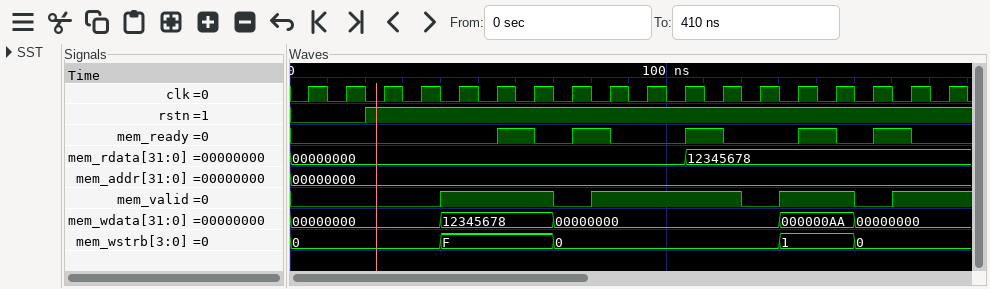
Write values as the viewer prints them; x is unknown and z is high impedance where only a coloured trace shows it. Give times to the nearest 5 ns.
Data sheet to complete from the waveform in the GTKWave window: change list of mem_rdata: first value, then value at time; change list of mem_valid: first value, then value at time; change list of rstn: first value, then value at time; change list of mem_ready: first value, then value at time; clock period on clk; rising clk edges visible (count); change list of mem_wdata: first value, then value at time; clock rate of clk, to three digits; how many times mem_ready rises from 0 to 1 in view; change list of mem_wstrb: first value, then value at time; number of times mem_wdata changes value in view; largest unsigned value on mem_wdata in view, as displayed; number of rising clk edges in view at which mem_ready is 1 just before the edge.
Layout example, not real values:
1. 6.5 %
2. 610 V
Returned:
1. 00000000, 12345678 at 105 ns
2. 0, 1 at 40 ns, 0 at 70 ns, 1 at 80 ns, 0 at 120 ns, 1 at 130 ns, 0 at 150 ns, 1 at 160 ns
3. 0, 1 at 20 ns
4. 0, 1 at 55 ns, 0 at 65 ns, 1 at 75 ns, 0 at 85 ns, 1 at 105 ns, 0 at 115 ns, 1 at 135 ns, 0 at 145 ns, 1 at 155 ns, 0 at 165 ns
5. 10 ns
6. 18
7. 00000000, 12345678 at 40 ns, 00000000 at 70 ns, 000000AA at 130 ns, 00000000 at 150 ns
8. 100 MHz
9. 5
10. 0, F at 40 ns, 0 at 70 ns, 1 at 130 ns, 0 at 150 ns
11. 4
12. 12345678
13. 5
